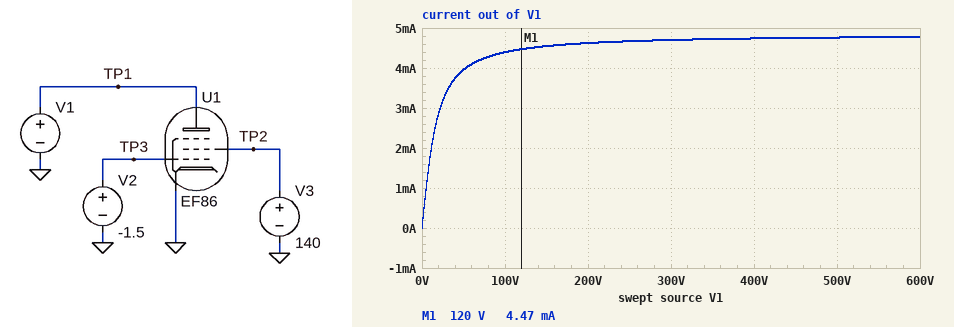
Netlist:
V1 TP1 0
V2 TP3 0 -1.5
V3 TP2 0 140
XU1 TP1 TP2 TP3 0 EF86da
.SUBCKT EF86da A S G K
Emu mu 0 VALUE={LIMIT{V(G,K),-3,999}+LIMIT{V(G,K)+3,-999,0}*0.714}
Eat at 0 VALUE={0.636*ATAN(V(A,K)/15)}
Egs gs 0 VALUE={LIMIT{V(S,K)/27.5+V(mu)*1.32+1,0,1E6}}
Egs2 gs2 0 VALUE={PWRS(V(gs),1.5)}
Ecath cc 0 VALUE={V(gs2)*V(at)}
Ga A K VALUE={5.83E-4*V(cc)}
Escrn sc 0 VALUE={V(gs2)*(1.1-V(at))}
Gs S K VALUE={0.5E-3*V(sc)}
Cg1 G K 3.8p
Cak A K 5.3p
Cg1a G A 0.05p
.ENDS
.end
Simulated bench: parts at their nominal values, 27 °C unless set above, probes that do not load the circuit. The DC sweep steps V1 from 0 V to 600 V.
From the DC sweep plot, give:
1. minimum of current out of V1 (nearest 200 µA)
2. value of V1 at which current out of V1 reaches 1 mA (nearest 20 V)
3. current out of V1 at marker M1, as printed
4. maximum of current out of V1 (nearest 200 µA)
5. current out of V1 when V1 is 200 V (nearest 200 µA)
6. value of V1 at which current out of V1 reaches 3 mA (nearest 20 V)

0 A
0 V
4.47 mA
4.8 mA
4.6 mA
20 V
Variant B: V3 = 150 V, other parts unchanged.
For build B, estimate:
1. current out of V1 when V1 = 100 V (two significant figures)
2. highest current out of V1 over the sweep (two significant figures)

5.0 mA
5.4 mA
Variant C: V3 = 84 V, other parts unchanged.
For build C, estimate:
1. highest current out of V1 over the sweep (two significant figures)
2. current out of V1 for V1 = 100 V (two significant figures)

1.7 mA
1.6 mA
